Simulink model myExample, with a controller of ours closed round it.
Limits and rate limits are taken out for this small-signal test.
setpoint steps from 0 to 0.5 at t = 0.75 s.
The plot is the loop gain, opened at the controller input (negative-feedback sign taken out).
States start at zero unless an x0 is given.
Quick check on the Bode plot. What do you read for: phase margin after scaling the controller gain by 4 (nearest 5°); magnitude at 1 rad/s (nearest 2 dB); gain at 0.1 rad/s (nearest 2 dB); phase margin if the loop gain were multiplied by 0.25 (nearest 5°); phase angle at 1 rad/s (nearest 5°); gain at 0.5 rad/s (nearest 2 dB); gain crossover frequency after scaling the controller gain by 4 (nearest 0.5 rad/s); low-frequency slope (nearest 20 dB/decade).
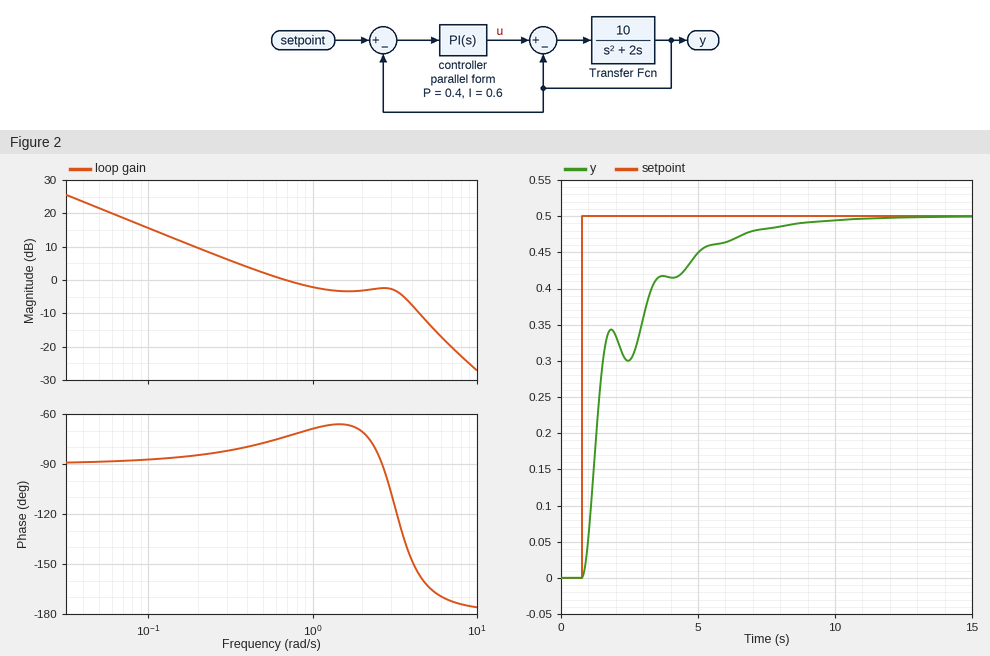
20°
-2 dB
16 dB
95°
-70°
2 dB
5.0 rad/s
-20 dB/decade
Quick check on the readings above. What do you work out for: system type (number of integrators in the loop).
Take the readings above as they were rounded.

1
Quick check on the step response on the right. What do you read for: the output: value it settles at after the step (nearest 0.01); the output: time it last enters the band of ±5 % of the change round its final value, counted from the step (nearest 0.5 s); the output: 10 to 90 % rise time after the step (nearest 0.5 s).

0.50
6.0 s
4.0 s
